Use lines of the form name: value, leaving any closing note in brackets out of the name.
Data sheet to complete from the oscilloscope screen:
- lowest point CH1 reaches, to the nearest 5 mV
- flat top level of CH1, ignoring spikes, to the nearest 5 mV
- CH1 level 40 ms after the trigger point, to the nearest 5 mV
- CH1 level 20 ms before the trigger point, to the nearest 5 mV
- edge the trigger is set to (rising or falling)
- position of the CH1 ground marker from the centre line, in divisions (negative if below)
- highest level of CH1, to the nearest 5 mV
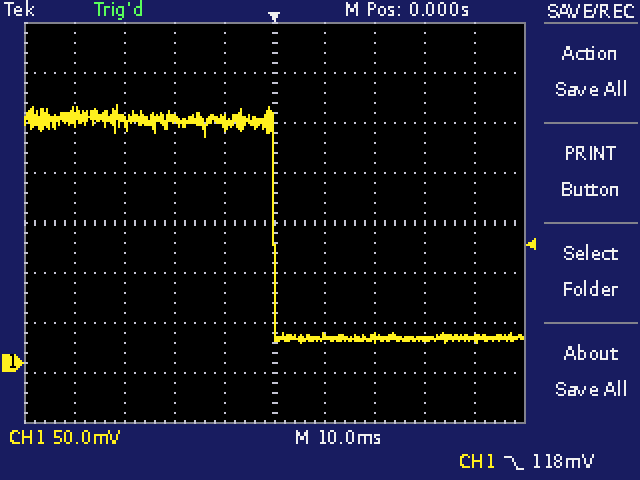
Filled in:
lowest point CH1 reaches, to the nearest 5 mV: 20 mV
flat top level of CH1, ignoring spikes, to the nearest 5 mV: 245 mV
CH1 level 40 ms after the trigger point, to the nearest 5 mV: 25 mV
CH1 level 20 ms before the trigger point, to the nearest 5 mV: 245 mV
edge the trigger is set to: falling
position of the CH1 ground marker from the centre line, in divisions: -2.8 div
highest level of CH1, to the nearest 5 mV: 260 mV
